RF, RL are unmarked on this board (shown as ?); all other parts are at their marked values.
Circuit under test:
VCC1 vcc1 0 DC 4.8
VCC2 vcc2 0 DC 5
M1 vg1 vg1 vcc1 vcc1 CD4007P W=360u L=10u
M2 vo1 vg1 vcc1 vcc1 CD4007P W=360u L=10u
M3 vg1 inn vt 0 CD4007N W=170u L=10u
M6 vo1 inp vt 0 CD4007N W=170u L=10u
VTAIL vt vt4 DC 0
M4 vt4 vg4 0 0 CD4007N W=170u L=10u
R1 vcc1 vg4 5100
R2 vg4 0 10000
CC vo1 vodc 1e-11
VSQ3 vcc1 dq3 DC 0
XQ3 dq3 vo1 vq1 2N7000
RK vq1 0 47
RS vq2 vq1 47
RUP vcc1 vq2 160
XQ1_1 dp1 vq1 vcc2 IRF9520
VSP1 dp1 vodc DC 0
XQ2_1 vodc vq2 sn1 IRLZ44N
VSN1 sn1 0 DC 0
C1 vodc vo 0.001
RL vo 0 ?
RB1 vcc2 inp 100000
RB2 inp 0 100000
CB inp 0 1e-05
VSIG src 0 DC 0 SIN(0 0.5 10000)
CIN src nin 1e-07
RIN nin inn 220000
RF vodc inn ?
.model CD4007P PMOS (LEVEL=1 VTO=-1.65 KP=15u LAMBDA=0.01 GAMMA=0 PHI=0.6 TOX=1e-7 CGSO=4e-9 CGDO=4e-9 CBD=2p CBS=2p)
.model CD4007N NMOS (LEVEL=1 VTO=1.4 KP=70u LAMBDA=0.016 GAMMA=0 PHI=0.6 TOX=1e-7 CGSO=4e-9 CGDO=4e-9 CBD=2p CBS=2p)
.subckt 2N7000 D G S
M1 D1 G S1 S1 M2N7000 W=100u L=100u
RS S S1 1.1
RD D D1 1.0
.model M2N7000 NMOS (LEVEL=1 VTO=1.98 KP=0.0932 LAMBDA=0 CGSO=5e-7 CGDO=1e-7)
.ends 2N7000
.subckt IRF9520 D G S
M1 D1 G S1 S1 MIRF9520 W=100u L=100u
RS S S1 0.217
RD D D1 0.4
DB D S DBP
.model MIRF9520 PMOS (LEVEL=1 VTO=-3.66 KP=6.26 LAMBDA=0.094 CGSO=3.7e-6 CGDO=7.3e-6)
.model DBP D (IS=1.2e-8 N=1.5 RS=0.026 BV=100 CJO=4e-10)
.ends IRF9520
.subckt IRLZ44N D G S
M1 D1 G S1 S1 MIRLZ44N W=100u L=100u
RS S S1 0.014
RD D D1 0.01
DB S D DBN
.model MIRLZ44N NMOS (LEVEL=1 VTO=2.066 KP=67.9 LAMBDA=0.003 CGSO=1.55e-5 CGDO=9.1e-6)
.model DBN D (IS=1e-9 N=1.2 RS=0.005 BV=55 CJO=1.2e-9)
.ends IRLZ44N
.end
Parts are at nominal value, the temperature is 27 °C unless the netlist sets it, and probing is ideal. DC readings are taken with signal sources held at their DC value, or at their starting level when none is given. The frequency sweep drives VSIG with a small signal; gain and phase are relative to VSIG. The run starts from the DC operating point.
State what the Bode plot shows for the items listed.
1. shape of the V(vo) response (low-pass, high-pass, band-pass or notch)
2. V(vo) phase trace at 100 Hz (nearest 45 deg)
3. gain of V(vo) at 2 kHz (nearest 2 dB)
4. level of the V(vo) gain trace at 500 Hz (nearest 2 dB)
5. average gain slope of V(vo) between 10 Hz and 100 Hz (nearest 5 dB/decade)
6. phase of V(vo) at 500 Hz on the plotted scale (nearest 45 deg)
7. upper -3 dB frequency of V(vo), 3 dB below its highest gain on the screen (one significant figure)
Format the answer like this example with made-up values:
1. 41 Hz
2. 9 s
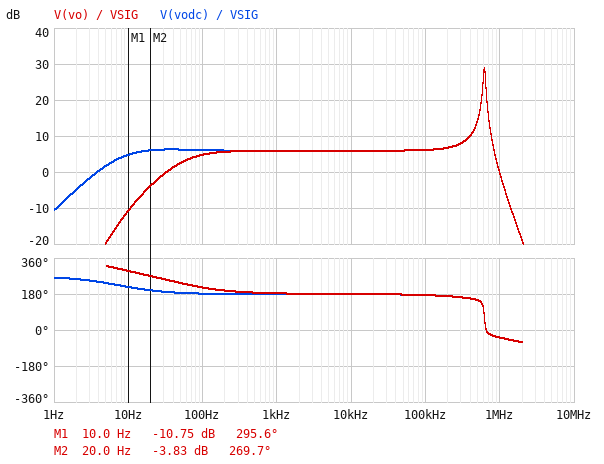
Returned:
1. band-pass
2. 225 deg
3. 6 dB
4. 6 dB
5. 15 dB/decade
6. 180 deg
7. 600 kHz
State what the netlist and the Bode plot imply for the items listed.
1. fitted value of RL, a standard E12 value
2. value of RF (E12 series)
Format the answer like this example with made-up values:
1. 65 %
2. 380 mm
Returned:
1. 2.7 Ω
2. 470 kΩ
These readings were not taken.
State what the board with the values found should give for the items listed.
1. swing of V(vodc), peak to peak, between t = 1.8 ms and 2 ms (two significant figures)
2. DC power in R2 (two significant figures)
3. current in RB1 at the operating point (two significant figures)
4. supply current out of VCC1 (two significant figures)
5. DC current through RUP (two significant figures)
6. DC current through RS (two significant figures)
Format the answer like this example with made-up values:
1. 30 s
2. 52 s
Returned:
1. 2.0 V
2. 1.0 mW
3. 25 µA
4. 28 mA
5. 17 mA
6. 17 mA
